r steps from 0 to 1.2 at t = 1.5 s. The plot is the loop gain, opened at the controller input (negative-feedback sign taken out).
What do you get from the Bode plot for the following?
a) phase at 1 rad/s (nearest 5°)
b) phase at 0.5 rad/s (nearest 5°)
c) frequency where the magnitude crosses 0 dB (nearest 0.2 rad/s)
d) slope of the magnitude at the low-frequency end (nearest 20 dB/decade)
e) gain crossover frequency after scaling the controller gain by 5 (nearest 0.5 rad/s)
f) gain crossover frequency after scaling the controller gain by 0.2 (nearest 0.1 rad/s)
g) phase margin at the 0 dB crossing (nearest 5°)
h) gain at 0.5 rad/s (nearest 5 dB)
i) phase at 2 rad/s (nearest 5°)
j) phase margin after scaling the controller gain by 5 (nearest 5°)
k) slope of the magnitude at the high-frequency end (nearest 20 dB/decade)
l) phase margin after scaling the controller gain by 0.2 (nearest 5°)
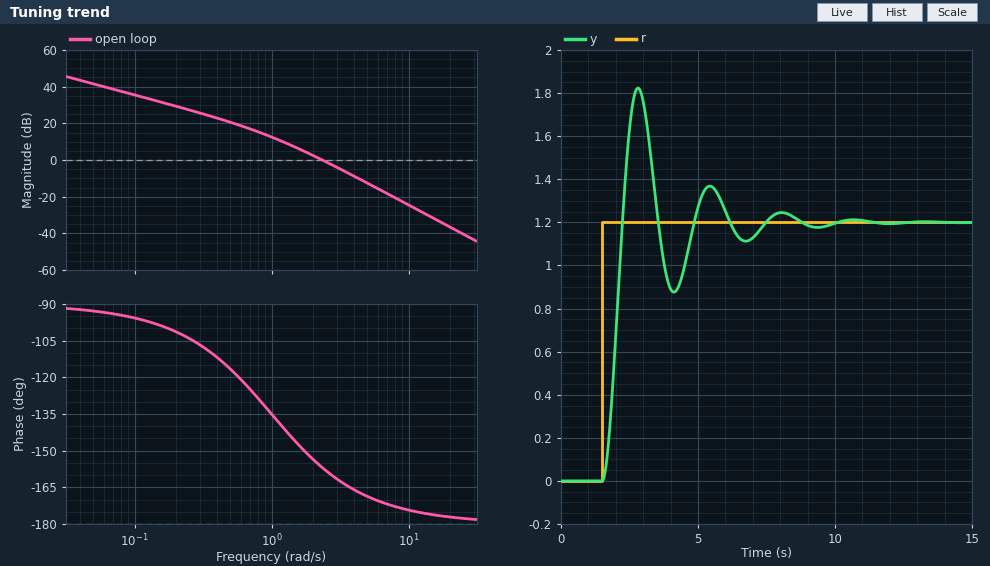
-135°
-115°
2.4 rad/s
-20 dB/decade
5.5 rad/s
0.9 rad/s
25°
20 dB
-155°
10°
-40 dB/decade
50°
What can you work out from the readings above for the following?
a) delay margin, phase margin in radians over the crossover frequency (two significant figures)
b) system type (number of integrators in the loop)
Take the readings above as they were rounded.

0.18 s
1
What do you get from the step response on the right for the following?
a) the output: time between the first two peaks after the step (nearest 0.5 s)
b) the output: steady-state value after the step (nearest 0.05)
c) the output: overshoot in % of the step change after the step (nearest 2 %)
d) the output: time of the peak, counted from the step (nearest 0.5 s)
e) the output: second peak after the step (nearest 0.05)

2.5 s
1.20
52 %
1.5 s
1.35
